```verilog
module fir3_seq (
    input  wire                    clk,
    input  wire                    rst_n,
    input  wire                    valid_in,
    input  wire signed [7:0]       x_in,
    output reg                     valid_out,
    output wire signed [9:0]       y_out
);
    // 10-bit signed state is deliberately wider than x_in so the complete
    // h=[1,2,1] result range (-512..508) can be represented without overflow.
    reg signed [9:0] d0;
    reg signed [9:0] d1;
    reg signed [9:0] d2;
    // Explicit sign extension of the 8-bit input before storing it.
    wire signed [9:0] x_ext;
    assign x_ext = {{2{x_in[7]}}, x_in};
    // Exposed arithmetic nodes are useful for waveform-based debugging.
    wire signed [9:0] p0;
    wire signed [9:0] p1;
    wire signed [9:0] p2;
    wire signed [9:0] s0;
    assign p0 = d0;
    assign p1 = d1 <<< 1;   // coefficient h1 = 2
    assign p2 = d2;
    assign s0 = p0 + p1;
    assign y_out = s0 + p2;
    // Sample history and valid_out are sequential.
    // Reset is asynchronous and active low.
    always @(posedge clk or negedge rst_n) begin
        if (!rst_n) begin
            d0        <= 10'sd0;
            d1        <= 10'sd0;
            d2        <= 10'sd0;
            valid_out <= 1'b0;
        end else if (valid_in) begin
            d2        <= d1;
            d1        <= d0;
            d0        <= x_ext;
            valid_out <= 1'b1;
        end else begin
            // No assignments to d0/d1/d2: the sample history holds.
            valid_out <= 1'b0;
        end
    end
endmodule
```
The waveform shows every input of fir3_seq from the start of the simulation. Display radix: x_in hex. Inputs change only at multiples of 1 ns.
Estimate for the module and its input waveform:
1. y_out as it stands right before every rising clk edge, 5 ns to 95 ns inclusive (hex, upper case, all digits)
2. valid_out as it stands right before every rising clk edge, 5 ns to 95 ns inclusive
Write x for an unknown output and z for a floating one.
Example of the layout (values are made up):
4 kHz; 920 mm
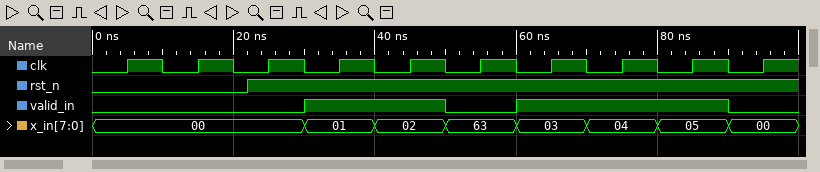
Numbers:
000, 000, 000, 000, 001, 004, 004, 008, 00C, 010; 0 0 0 0 1 1 0 1 1 1
